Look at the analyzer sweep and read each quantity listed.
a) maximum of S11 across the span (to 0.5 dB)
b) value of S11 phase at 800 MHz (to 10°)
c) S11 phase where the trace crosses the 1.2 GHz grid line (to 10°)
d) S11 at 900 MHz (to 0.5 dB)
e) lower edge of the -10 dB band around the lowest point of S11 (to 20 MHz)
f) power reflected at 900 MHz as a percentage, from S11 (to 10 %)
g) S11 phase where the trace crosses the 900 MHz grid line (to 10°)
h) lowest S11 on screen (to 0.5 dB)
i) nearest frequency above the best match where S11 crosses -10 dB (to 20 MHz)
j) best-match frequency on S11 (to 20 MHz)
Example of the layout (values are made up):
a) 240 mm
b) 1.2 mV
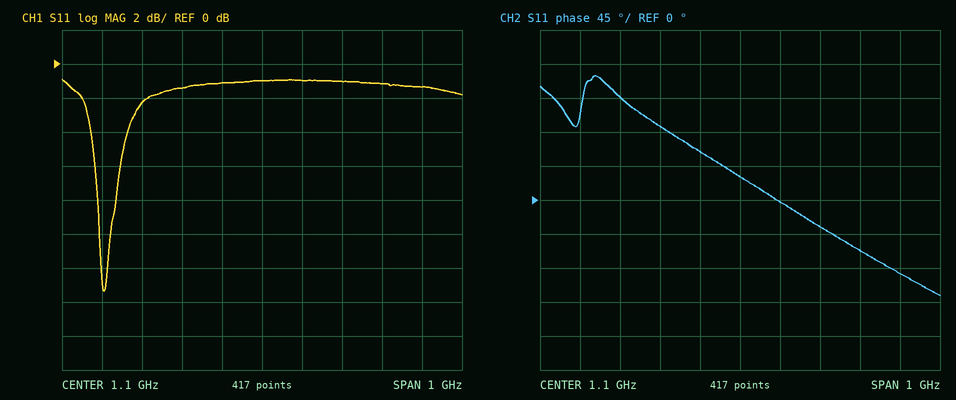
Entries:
a) -1.0 dB
b) 140°
c) 0°
d) -1.5 dB
e) 700 MHz
f) 70 %
g) 100°
h) -13.5 dB
i) 720 MHz
j) 700 MHz
